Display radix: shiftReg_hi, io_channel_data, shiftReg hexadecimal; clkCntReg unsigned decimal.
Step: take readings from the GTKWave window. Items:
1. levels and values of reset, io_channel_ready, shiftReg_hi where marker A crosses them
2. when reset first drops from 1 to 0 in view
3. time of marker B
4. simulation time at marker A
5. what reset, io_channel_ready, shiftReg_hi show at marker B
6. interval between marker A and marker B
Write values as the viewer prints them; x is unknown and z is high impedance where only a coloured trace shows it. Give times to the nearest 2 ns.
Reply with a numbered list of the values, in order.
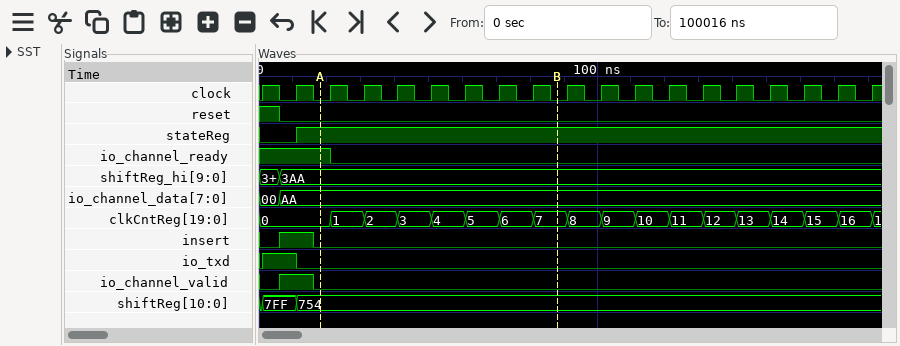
1. reset=0, io_channel_ready=1, shiftReg_hi=3AA
2. 6 ns
3. 88 ns
4. 18 ns
5. reset=0, io_channel_ready=0, shiftReg_hi=3AA
6. 70 ns
